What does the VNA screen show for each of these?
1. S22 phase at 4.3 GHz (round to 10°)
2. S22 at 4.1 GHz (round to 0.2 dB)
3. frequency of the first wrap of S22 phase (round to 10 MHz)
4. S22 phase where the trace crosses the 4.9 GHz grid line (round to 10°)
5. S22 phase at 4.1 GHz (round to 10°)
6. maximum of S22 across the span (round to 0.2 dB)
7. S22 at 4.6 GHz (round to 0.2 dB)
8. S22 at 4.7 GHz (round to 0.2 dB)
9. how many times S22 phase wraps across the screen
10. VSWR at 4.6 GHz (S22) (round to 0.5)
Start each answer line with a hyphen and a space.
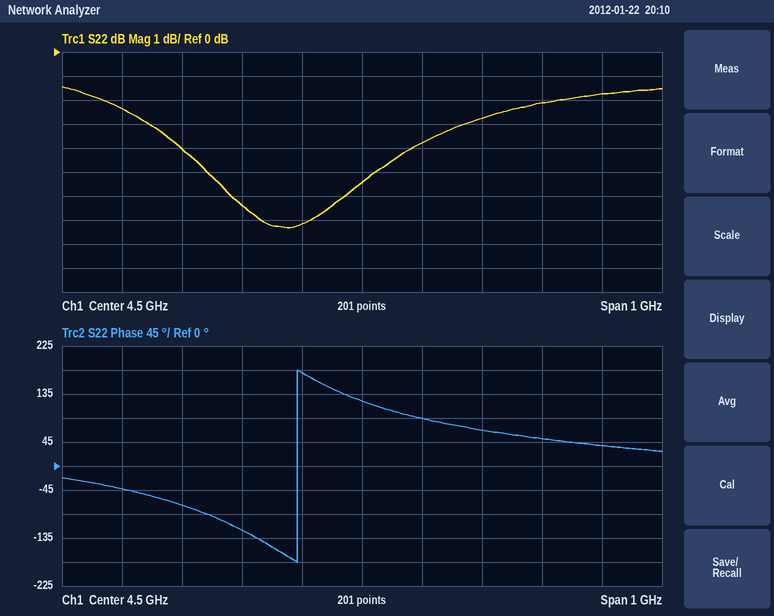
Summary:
- -120°
- -2.4 dB
- 4.39 GHz
- 40°
- -40°
- -1.4 dB
- -3.8 dB
- -2.8 dB
- 1
- 4.5
